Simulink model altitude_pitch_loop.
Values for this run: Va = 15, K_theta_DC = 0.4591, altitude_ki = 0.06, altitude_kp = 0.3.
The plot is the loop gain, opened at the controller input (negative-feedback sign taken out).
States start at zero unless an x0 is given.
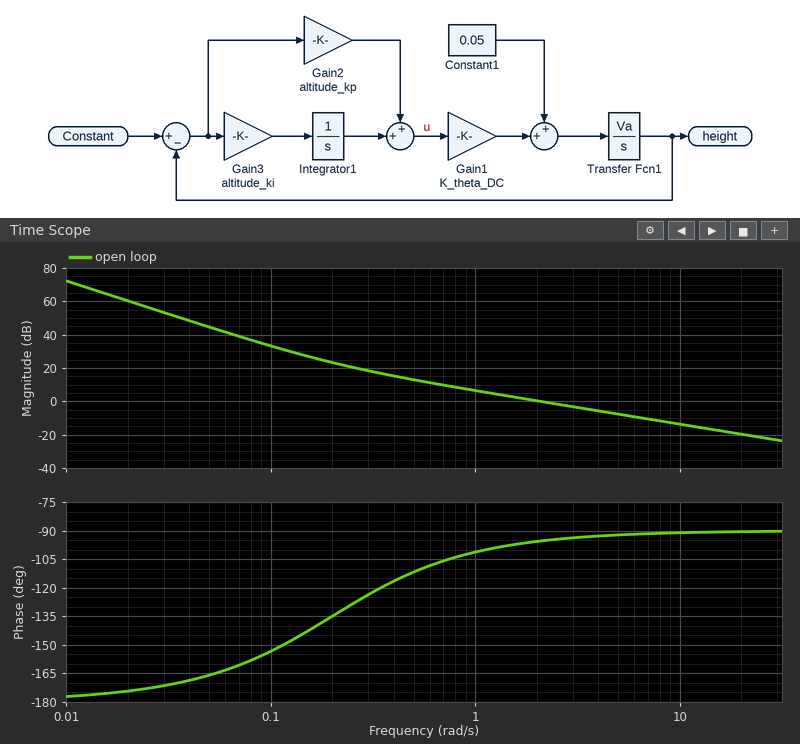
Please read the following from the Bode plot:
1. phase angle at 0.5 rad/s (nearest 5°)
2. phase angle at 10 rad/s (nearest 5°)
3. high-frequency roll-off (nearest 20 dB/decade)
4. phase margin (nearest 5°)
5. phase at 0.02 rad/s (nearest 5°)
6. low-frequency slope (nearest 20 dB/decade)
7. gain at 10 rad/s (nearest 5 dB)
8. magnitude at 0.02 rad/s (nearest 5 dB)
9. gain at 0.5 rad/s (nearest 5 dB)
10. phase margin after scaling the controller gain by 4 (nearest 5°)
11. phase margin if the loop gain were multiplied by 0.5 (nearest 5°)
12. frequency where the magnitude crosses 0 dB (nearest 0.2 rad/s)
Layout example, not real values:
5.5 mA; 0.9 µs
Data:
-110°; -90°; -20 dB/decade; 85°; -175°; -40 dB/decade; -15 dB; 60 dB; 15 dB; 90°; 80°; 2.0 rad/s
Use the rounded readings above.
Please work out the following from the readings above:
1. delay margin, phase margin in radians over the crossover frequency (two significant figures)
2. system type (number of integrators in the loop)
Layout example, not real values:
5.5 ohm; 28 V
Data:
0.74 s; 2
